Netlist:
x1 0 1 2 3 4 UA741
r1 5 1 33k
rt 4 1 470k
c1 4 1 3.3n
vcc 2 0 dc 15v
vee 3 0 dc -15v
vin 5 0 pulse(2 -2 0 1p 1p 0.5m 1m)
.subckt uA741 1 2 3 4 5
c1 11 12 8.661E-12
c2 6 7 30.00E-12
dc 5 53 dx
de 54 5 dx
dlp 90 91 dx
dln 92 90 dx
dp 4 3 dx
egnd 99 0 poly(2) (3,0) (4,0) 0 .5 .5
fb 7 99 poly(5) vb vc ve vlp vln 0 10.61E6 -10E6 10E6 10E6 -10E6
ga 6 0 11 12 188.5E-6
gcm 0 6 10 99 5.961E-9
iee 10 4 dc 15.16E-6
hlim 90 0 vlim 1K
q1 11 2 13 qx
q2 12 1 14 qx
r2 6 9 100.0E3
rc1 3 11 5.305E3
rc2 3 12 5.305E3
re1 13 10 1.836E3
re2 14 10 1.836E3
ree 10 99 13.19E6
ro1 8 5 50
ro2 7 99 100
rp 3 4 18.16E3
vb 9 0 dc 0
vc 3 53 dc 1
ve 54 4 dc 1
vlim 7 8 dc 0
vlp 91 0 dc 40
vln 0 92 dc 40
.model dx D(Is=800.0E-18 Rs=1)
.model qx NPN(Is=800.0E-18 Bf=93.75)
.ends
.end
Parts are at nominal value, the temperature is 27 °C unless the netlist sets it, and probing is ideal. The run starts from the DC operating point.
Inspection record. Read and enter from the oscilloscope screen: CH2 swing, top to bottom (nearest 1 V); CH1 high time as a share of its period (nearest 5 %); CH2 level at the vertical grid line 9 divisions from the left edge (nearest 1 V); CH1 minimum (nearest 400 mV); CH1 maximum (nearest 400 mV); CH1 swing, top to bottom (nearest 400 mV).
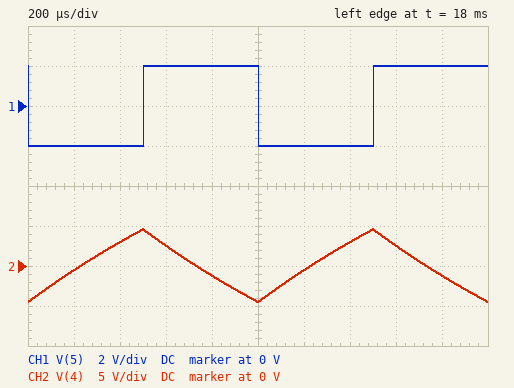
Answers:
9 V
50 %
-1 V
-2.0 V
2.0 V
4.0 V
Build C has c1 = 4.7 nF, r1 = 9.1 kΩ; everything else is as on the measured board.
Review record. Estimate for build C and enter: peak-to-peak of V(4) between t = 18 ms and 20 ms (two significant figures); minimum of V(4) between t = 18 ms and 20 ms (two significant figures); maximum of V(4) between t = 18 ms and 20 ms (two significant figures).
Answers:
23 V
-12 V
12 V
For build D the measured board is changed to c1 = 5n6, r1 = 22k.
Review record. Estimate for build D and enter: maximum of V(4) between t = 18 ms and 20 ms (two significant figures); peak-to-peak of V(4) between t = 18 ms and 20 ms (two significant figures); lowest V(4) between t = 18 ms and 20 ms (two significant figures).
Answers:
4.1 V
8.1 V
-4.0 V
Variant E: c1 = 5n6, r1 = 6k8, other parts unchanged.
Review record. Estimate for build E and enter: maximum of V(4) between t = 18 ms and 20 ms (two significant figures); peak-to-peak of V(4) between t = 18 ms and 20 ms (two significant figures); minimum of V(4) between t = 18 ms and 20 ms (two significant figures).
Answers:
13 V
26 V
-13 V
